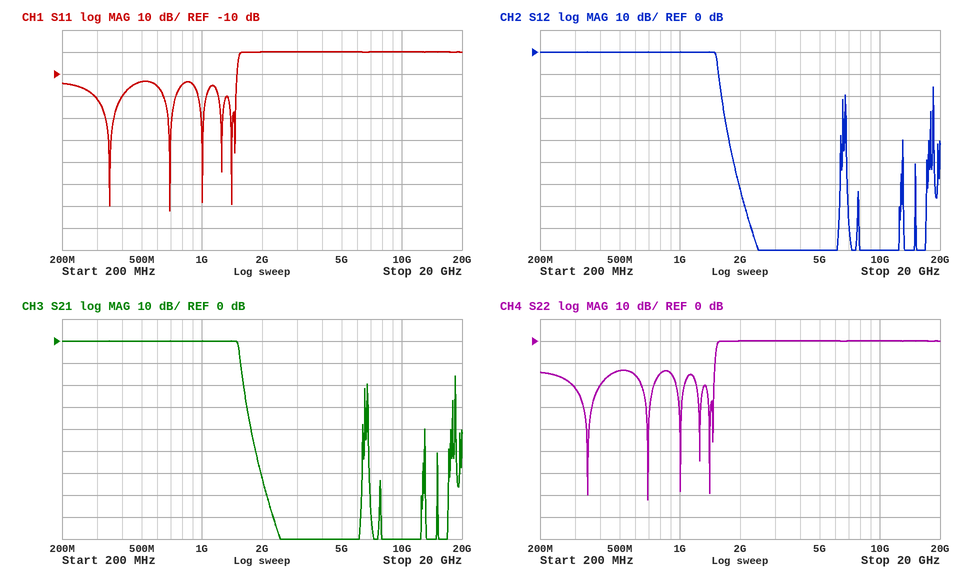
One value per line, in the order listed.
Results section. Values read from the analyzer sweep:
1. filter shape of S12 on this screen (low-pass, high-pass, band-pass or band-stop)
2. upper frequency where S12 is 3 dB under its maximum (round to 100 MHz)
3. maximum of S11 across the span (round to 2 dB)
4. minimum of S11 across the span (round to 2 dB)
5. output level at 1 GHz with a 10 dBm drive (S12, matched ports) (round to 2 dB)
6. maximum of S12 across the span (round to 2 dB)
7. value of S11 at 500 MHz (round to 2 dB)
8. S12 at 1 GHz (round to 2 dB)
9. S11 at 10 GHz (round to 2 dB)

low-pass
1.5 GHz
0 dB
-72 dB
10 dBm
0 dB
-14 dB
0 dB
0 dB
